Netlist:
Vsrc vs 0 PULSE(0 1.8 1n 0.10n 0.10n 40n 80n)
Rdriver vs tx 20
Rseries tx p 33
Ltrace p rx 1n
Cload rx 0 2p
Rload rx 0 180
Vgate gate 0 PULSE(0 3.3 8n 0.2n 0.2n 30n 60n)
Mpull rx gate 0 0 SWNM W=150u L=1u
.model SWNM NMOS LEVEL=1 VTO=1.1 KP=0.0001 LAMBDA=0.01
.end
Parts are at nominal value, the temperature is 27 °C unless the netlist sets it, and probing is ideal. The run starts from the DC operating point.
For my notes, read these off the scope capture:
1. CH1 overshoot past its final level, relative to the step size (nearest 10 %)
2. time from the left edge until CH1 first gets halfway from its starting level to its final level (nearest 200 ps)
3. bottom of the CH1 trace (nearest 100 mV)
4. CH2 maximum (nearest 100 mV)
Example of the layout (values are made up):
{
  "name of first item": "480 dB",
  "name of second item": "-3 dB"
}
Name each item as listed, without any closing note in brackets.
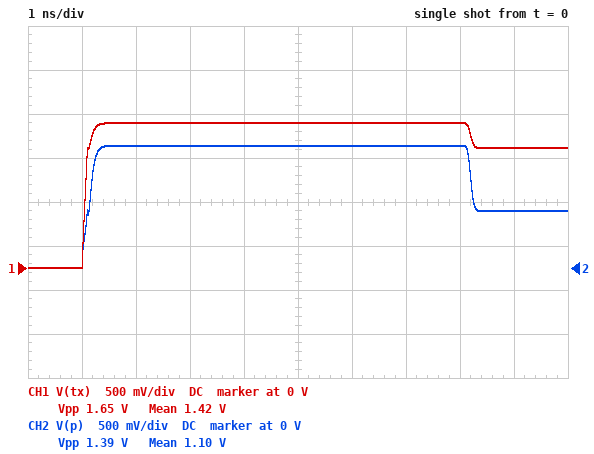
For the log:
{
  "CH1 overshoot past its final level, relative to the step size": "20 %",
  "time from the left edge until CH1 first gets halfway from its starting level to its final level": "1.0 ns",
  "bottom of the CH1 trace": "0 V",
  "CH2 maximum": "1.4 V"
}
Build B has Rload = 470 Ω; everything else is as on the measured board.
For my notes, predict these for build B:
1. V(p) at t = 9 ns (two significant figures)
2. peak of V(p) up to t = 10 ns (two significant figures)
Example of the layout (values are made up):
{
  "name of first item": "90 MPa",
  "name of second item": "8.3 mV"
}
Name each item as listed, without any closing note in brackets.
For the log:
{
  "V(p) at t = 9 ns": "690 mV",
  "peak of V(p) up to t = 10 ns": "1.6 V"
}
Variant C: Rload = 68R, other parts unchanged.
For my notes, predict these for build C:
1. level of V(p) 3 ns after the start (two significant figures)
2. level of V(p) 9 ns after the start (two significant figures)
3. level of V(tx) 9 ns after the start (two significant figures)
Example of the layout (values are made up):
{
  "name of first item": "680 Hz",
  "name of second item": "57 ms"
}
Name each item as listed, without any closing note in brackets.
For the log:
{
  "level of V(p) 3 ns after the start": "1.0 V",
  "level of V(p) 9 ns after the start": "540 mV",
  "level of V(tx) 9 ns after the start": "1.3 V"
}
